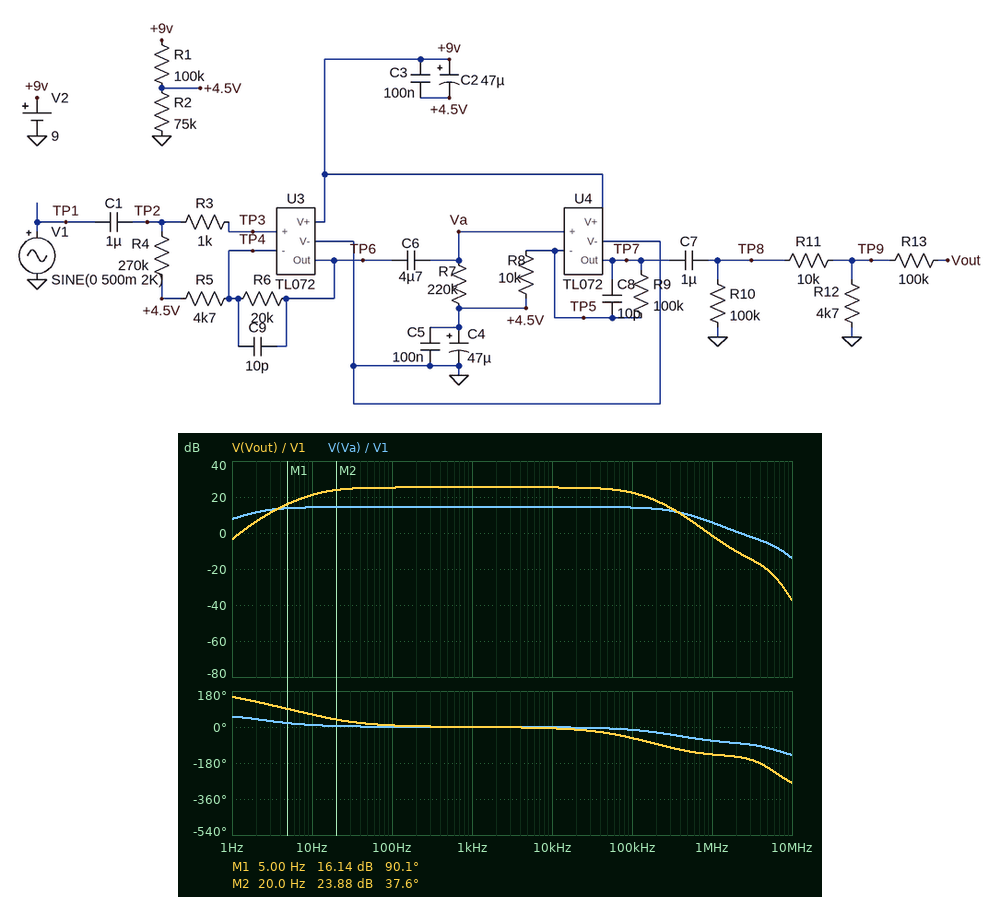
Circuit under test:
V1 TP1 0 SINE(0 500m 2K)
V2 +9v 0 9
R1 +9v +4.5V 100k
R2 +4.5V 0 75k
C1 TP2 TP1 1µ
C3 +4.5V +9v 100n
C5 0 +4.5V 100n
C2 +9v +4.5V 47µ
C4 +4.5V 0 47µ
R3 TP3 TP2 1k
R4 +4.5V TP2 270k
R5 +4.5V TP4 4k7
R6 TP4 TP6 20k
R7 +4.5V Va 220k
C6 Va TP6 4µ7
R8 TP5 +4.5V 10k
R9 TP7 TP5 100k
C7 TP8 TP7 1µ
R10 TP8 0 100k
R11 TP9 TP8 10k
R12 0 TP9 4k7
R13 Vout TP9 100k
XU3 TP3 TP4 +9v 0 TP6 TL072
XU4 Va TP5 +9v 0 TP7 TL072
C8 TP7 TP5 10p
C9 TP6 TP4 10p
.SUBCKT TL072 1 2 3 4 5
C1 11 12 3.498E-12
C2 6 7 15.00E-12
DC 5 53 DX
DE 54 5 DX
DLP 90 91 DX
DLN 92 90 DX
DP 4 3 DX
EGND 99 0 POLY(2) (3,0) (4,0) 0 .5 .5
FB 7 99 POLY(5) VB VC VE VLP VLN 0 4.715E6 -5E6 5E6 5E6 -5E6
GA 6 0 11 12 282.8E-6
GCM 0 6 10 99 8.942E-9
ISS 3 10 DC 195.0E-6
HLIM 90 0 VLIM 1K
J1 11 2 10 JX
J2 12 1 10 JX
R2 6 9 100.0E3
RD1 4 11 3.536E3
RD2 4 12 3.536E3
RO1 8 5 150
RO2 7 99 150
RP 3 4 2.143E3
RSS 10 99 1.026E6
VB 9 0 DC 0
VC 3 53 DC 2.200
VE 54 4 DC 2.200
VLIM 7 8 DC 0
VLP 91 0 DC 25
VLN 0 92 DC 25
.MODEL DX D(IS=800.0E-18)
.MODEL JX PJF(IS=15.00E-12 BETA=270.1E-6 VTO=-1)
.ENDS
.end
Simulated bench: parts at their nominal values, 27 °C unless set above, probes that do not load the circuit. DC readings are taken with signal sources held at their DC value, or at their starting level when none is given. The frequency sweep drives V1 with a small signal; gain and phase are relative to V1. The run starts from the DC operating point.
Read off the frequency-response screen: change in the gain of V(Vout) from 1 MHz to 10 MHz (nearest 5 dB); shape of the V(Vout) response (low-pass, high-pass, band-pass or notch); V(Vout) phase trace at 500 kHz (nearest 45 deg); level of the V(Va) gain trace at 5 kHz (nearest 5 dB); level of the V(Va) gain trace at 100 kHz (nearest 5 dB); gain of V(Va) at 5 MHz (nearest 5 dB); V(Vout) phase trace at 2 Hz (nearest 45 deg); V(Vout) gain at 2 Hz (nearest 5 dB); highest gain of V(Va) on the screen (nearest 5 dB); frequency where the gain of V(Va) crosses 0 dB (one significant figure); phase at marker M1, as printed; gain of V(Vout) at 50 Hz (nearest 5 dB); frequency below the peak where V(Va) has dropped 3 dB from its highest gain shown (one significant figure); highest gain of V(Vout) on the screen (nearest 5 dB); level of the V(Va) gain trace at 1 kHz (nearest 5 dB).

-35 dB
band-pass
-135 deg
15 dB
15 dB
-5 dB
135 deg
5 dB
15 dB
2 MHz
90.1 deg
25 dB
2 Hz
25 dB
15 dB
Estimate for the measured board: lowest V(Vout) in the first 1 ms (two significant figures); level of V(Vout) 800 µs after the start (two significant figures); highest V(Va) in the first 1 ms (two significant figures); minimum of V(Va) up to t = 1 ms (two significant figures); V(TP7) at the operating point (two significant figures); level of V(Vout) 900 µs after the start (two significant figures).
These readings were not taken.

-770 mV
-770 mV
6.5 V
1.6 V
3.9 V
-770 mV
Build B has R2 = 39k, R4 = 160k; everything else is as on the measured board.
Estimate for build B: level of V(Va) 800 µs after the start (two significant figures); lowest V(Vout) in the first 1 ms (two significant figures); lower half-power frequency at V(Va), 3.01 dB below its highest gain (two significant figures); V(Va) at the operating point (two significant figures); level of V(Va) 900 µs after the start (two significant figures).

1.6 V
-370 mV
2.4 Hz
2.5 V
1.5 V
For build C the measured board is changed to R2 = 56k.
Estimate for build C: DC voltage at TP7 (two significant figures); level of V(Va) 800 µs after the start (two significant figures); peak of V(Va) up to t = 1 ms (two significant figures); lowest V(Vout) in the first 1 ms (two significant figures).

3.2 V
1.7 V
5.9 V
-580 mV
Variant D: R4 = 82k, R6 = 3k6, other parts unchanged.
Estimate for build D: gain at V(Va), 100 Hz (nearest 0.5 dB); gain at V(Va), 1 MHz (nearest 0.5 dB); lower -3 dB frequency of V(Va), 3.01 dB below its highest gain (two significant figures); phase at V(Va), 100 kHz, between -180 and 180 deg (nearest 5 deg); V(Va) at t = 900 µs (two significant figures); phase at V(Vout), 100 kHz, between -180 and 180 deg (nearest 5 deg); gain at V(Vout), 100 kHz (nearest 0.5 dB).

5.0 dB
4.0 dB
2.6 Hz
-5 deg
3.0 V
-45 deg
13.0 dB
